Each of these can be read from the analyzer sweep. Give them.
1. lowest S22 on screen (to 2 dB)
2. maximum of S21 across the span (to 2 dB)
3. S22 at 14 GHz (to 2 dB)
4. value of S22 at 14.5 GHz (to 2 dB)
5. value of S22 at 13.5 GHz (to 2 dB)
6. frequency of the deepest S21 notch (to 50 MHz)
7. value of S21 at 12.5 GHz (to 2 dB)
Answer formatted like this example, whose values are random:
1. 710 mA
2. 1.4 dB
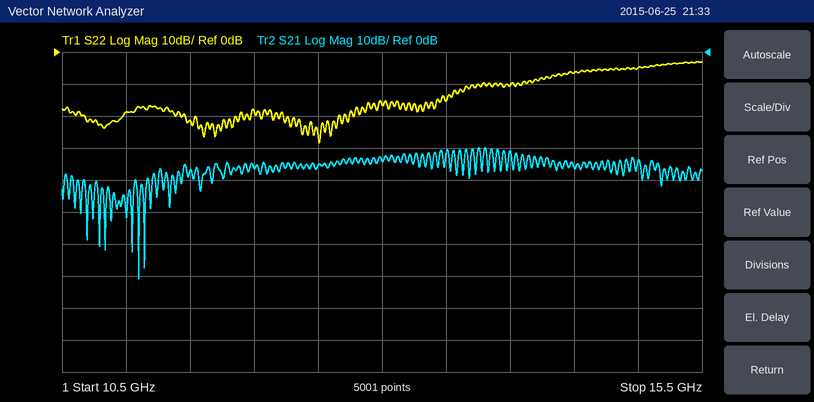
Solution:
1. -28 dB
2. -30 dB
3. -10 dB
4. -6 dB
5. -16 dB
6. 11.10 GHz
7. -36 dB
